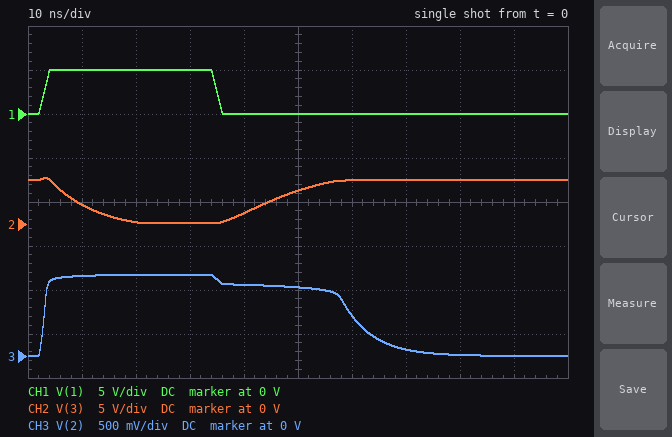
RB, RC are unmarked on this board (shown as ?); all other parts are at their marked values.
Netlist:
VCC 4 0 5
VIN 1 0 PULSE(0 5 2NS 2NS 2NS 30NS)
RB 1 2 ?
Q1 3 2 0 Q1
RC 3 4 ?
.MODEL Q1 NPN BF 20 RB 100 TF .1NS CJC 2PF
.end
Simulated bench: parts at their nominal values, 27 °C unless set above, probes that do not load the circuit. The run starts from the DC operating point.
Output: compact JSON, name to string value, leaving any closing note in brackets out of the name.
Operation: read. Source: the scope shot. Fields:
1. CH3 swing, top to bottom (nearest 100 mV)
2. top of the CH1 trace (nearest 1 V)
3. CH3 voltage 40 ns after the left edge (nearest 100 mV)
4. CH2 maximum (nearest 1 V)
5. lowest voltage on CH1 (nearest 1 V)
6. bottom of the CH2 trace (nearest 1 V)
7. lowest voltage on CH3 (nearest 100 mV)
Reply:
{"CH3 swing, top to bottom": "900 mV", "top of the CH1 trace": "5 V", "CH3 voltage 40 ns after the left edge": "800 mV", "CH2 maximum": "5 V", "lowest voltage on CH1": "0 V", "bottom of the CH2 trace": "0 V", "lowest voltage on CH3": "0 V"}
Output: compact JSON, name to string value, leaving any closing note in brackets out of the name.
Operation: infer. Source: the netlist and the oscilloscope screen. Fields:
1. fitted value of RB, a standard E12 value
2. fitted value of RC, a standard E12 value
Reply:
{"fitted value of RB, a standard E12 value": "4.7 kΩ", "fitted value of RC, a standard E12 value": "470 Ω"}
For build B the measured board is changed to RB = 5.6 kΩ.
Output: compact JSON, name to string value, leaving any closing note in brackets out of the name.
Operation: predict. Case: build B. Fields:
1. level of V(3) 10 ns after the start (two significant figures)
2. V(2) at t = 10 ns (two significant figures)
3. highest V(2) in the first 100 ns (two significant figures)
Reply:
{"level of V(3) 10 ns after the start": "2.6 V", "V(2) at t = 10 ns": "890 mV", "highest V(2) in the first 100 ns": "910 mV"}
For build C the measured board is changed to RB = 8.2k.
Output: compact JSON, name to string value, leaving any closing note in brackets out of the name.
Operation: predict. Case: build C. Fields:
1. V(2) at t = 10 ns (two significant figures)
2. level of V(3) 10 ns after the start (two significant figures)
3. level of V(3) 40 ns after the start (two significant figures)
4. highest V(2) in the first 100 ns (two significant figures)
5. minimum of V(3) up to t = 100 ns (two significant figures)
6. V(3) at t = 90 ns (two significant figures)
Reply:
{"V(2) at t = 10 ns": "860 mV", "level of V(3) 10 ns after the start": "3.4 V", "level of V(3) 40 ns after the start": "2.2 V", "highest V(2) in the first 100 ns": "880 mV", "minimum of V(3) up to t = 100 ns": "1.0 V", "V(3) at t = 90 ns": "5.0 V"}
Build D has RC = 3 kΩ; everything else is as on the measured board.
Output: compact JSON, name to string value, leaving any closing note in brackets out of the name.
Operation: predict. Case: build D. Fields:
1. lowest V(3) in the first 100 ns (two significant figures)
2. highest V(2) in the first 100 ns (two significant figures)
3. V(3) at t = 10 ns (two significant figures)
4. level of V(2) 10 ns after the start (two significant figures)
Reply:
{"lowest V(3) in the first 100 ns": "38 mV", "highest V(2) in the first 100 ns": "890 mV", "V(3) at t = 10 ns": "1.4 V", "level of V(2) 10 ns after the start": "880 mV"}
